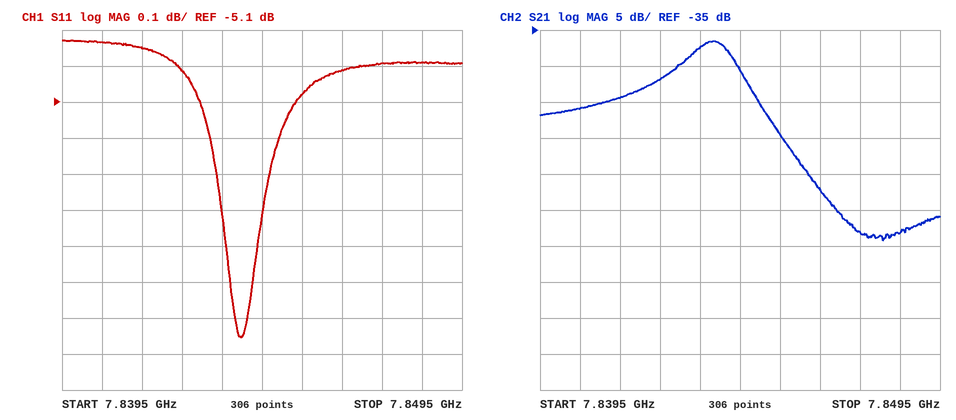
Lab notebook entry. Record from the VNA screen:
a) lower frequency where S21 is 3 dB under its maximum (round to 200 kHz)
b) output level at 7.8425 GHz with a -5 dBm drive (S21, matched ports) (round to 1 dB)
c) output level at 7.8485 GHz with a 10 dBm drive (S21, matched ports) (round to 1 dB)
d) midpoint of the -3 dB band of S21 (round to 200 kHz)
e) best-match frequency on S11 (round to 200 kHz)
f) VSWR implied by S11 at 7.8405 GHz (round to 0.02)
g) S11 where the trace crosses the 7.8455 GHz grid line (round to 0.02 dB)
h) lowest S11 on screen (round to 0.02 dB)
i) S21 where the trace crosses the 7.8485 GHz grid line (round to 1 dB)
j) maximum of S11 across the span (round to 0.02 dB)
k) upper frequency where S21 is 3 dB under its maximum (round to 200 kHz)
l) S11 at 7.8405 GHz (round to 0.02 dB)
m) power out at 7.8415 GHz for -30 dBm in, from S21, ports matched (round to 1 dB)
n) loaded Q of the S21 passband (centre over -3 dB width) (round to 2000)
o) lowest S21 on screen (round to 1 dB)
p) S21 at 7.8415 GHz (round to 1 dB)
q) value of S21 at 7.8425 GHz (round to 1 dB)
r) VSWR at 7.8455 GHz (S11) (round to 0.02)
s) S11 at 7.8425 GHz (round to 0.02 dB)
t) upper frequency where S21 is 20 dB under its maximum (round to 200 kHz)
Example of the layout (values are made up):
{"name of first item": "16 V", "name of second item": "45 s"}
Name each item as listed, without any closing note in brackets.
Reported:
{"lower frequency where S21 is 3 dB under its maximum": "7.8430 GHz", "output level at 7.8425 GHz with a -5 dBm drive (S21, matched ports)": "-47 dBm", "output level at 7.8485 GHz with a 10 dBm drive (S21, matched ports)": "-53 dBm", "midpoint of the -3 dB band of S21": "7.8438 GHz", "best-match frequency on S11": "7.8440 GHz", "VSWR implied by S11 at 7.8405 GHz": "3.62", "S11 where the trace crosses the 7.8455 GHz grid line": "-5.08 dB", "lowest S11 on screen": "-5.76 dB", "S21 where the trace crosses the 7.8485 GHz grid line": "-63 dB", "maximum of S11 across the span": "-4.92 dB", "upper frequency where S21 is 3 dB under its maximum": "7.8444 GHz", "S11 at 7.8405 GHz": "-4.94 dB", "power out at 7.8415 GHz for -30 dBm in, from S21, ports matched": "-74 dBm", "loaded Q of the S21 passband (centre over -3 dB width)": "6000", "lowest S21 on screen": "-64 dB", "S21 at 7.8415 GHz": "-44 dB", "value of S21 at 7.8425 GHz": "-42 dB", "VSWR at 7.8455 GHz (S11)": "3.52", "S11 at 7.8425 GHz": "-5.02 dB", "upper frequency where S21 is 20 dB under its maximum": "7.8464 GHz"}
